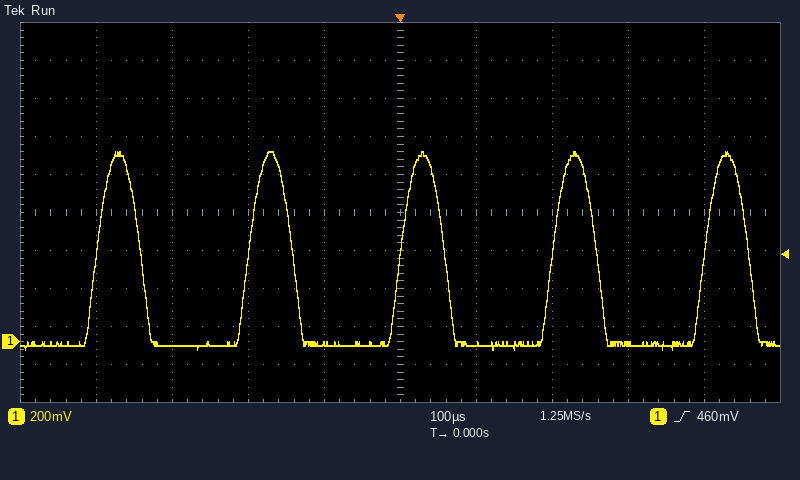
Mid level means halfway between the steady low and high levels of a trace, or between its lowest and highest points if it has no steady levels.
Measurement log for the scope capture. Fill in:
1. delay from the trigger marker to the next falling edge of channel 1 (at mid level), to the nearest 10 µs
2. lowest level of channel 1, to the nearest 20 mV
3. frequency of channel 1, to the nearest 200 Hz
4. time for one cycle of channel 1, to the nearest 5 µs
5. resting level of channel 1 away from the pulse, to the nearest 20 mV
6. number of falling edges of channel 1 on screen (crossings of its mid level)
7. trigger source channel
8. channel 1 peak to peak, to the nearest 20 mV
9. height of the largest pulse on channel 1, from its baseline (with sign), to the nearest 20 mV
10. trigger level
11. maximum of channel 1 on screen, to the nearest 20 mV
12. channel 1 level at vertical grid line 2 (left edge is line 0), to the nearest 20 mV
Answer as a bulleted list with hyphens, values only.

- 60 µs
- -40 mV
- 5.0 kHz
- 200 µs
- -20 mV
- 5
- channel 1
- 1.04 V
- +1.02 V
- 460 mV
- 1.00 V
- -20 mV
